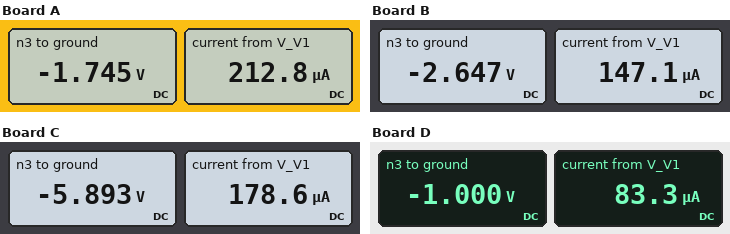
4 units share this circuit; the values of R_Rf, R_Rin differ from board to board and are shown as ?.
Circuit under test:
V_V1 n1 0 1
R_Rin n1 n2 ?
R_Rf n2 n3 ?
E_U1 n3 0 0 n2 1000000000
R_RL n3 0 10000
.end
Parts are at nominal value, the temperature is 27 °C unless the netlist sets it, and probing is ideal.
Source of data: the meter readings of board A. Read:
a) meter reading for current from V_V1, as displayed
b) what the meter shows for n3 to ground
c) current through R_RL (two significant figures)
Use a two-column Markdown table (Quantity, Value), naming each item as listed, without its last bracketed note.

| Quantity | Value |
|---|---|
| meter reading for current from V_V1, as displayed | 212.8 µA |
| what the meter shows for n3 to ground | -1.745 V |
| current through R_RL | 170 µA |
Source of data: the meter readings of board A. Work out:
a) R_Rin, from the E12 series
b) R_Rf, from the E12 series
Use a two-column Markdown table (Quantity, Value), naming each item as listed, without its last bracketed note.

| Quantity | Value |
|---|---|
| R_Rin, from the E12 series | 4.7 kΩ |
| R_Rf, from the E12 series | 8.2 kΩ |
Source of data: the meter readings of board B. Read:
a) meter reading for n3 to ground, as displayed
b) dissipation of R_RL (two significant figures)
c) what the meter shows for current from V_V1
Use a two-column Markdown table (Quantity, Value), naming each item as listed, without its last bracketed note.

| Quantity | Value |
|---|---|
| meter reading for n3 to ground, as displayed | -2.647 V |
| dissipation of R_RL | 700 µW |
| what the meter shows for current from V_V1 | 147.1 µA |
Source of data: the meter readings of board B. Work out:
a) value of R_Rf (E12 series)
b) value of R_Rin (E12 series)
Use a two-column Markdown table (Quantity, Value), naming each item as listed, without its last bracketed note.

| Quantity | Value |
|---|---|
| value of R_Rf | 18 kΩ |
| value of R_Rin | 6.8 kΩ |
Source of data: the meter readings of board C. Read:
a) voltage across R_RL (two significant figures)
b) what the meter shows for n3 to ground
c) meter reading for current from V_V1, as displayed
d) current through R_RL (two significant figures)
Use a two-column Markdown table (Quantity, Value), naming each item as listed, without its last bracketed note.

| Quantity | Value |
|---|---|
| voltage across R_RL | 5.9 V |
| what the meter shows for n3 to ground | -5.893 V |
| meter reading for current from V_V1, as displayed | 178.6 µA |
| current through R_RL | 590 µA |
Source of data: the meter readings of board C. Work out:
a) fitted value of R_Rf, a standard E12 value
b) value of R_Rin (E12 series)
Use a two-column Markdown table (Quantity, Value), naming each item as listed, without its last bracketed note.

| Quantity | Value |
|---|---|
| fitted value of R_Rf, a standard E12 value | 33 kΩ |
| value of R_Rin | 5.6 kΩ |
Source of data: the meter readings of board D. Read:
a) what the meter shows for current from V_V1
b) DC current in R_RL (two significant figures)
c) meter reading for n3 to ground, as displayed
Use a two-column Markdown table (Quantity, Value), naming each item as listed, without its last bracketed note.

| Quantity | Value |
|---|---|
| what the meter shows for current from V_V1 | 83.3 µA |
| DC current in R_RL | 100 µA |
| meter reading for n3 to ground, as displayed | -1.000 V |
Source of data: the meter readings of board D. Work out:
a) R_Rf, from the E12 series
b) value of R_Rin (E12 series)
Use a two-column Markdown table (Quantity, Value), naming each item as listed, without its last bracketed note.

| Quantity | Value |
|---|---|
| R_Rf, from the E12 series | 12 kΩ |
| value of R_Rin | 12 kΩ |
